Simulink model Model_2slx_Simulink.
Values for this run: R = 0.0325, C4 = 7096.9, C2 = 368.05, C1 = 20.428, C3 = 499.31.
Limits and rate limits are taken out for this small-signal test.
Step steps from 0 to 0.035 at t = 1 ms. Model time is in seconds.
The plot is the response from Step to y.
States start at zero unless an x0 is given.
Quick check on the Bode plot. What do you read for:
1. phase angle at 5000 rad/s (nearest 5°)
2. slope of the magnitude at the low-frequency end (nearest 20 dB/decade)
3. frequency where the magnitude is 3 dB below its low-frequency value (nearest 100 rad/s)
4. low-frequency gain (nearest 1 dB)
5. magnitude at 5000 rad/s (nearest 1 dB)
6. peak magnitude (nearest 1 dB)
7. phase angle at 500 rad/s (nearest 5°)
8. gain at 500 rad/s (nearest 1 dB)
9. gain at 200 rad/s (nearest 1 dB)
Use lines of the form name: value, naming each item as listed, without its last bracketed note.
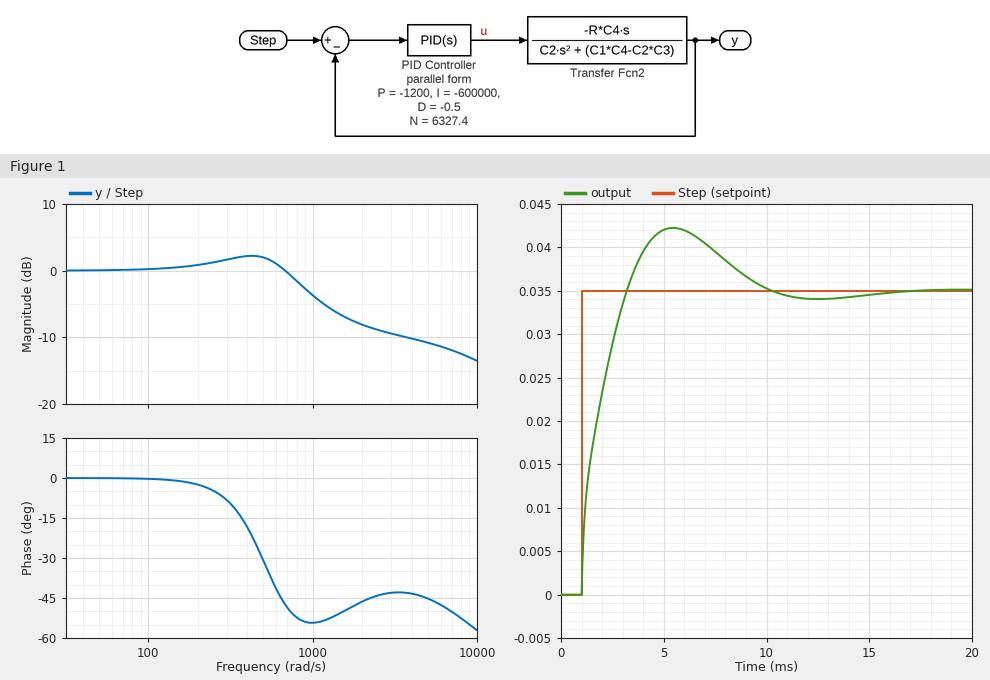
phase angle at 5000 rad/s: -45°
slope of the magnitude at the low-frequency end: 0 dB/decade
frequency where the magnitude is 3 dB below its low-frequency value: 900 rad/s
low-frequency gain: 0 dB
magnitude at 5000 rad/s: -11 dB
peak magnitude: 2 dB
phase angle at 500 rad/s: -30°
gain at 500 rad/s: 2 dB
gain at 200 rad/s: 1 dB
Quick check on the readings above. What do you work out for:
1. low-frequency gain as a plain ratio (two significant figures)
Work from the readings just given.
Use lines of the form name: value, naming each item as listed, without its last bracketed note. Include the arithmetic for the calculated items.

low-frequency gain as a plain ratio: 10^(0 / 20) = 1.0
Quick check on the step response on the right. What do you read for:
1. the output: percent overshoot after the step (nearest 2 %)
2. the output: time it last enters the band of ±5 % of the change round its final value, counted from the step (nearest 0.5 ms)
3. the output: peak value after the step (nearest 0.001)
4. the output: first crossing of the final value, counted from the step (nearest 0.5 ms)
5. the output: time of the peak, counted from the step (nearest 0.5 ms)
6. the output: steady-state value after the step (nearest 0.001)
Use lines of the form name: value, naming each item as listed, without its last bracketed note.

the output: percent overshoot after the step: 20 %
the output: time it last enters the band of ±5 % of the change round its final value, counted from the step: 8.0 ms
the output: peak value after the step: 0.042
the output: first crossing of the final value, counted from the step: 2.0 ms
the output: time of the peak, counted from the step: 4.5 ms
the output: steady-state value after the step: 0.035
